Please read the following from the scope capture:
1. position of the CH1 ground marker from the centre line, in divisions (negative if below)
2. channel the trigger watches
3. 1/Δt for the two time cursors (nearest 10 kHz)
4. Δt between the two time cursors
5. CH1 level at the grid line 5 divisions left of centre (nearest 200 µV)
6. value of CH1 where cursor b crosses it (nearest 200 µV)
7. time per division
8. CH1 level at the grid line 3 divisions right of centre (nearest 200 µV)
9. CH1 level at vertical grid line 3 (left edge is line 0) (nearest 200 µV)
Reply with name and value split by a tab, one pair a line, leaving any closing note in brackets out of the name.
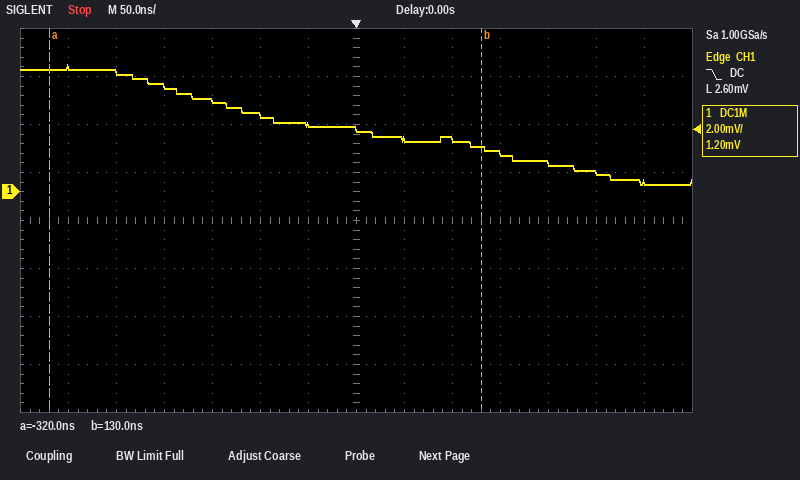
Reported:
position of the CH1 ground marker from the centre line, in divisions	+0.6 div
channel the trigger watches	CH1
1/Δt for the two time cursors	2.22 MHz
Δt between the two time cursors	450 ns
CH1 level at the grid line 5 divisions left of centre	5.0 mV
value of CH1 where cursor b crosses it	1.8 mV
time per division	50 ns
CH1 level at the grid line 3 divisions right of centre	1.6 mV
CH1 level at vertical grid line 3 (left edge is line 0)	4.4 mV
